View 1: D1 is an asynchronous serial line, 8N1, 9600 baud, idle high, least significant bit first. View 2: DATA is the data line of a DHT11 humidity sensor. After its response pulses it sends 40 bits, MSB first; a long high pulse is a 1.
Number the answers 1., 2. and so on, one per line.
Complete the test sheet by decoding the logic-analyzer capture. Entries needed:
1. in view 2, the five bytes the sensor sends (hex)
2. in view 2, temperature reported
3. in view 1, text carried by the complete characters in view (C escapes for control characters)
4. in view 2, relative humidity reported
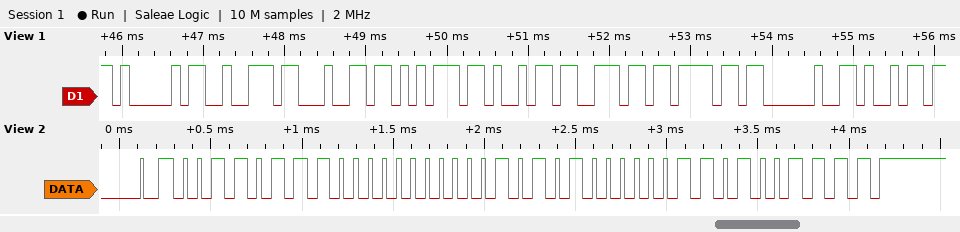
1. 37 00 15 03 4F
2. 21.3 °C
3. "Arduino i"
4. 55 %
